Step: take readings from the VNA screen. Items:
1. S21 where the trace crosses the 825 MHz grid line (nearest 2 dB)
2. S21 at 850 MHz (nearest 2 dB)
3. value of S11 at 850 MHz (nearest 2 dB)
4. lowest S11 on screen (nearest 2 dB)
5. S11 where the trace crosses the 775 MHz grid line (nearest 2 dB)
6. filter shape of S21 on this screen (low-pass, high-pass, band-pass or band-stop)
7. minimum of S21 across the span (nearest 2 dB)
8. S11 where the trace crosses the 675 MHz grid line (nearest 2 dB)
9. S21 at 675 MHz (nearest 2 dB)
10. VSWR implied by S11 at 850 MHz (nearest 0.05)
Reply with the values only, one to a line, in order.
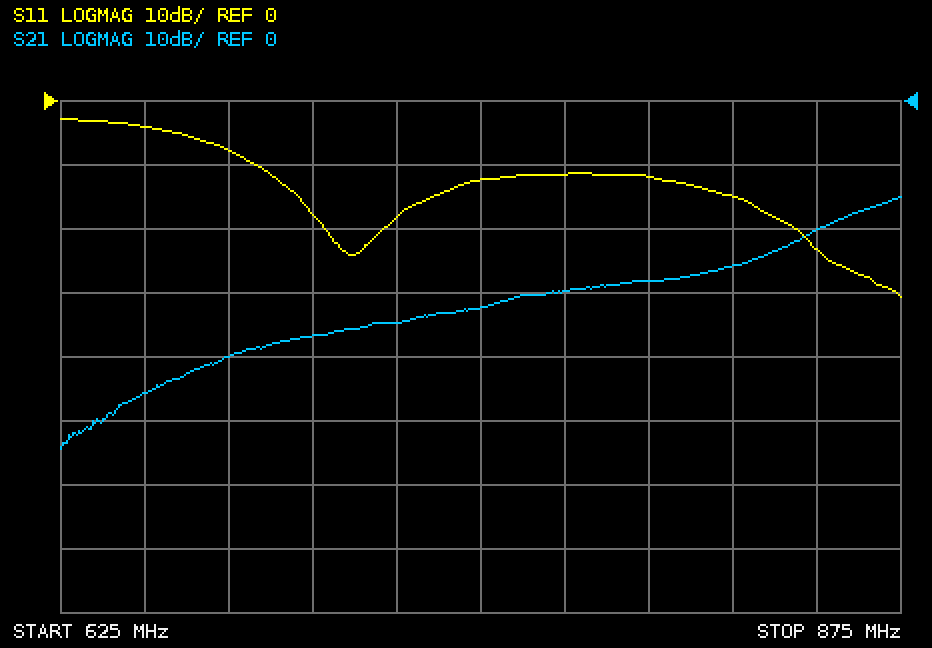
-26 dB
-20 dB
-24 dB
-30 dB
-12 dB
high-pass
-54 dB
-8 dB
-40 dB
1.15
